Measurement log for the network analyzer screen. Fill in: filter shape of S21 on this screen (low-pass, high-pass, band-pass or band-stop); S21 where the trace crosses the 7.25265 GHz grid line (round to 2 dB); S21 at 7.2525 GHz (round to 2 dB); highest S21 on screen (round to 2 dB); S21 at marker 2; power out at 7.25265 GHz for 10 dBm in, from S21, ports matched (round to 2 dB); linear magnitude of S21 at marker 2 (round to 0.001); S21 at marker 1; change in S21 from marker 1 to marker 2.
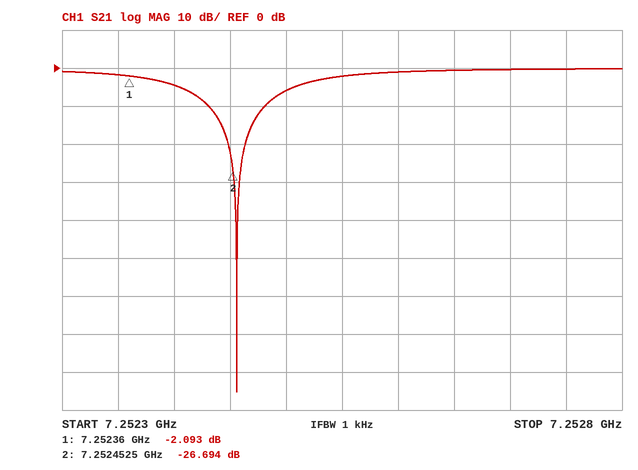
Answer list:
band-stop
0 dB
-6 dB
0 dB
-26.694 dB
10 dBm
0.046
-2.093 dB
-24.601 dB
